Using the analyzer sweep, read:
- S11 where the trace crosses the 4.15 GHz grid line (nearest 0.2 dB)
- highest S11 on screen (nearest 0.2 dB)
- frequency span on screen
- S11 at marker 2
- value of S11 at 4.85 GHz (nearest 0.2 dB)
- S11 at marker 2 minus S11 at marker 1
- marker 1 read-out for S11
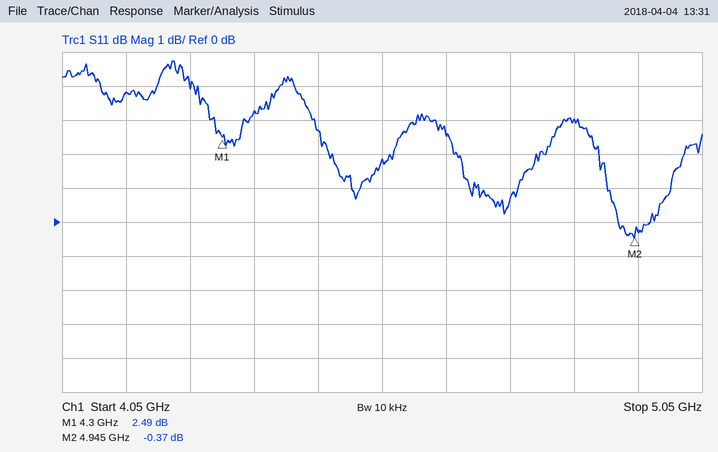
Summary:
3.8 dB
4.8 dB
1 GHz
-0.37 dB
3.0 dB
-2.86 dB
2.49 dB
